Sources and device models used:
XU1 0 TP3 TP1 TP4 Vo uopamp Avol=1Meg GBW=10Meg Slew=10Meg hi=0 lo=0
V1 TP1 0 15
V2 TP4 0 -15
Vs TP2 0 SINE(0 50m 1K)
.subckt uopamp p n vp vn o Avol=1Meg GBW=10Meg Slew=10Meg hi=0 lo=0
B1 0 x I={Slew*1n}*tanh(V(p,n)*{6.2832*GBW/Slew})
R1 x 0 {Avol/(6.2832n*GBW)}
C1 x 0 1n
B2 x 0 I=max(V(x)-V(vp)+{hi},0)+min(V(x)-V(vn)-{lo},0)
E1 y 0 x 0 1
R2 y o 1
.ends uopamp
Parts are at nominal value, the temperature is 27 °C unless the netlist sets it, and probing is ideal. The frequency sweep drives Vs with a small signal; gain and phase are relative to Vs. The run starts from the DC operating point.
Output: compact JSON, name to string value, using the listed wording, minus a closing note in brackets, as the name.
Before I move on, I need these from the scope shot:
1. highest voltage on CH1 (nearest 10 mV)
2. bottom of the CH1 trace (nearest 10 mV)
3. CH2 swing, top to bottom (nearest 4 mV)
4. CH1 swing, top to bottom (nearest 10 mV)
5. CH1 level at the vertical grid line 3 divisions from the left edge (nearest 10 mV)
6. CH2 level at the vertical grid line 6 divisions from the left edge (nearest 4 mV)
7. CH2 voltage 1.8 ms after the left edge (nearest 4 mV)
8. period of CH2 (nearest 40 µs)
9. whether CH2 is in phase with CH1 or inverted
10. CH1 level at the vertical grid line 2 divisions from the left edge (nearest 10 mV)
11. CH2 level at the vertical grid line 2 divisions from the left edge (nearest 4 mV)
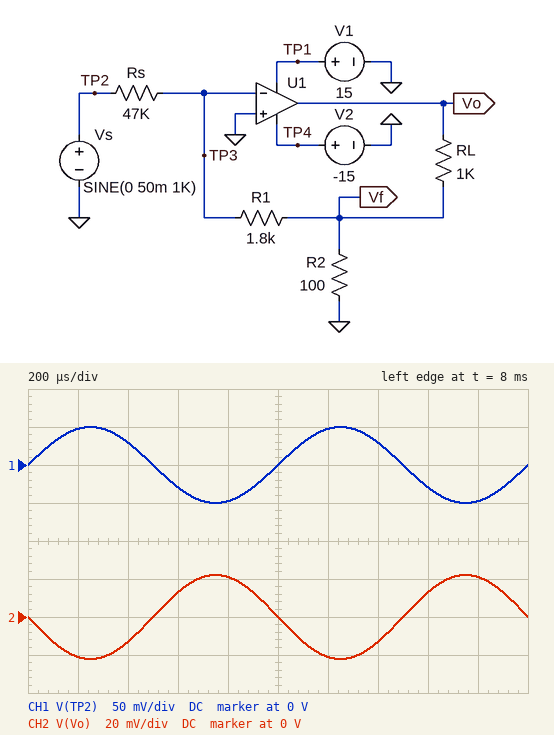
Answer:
{"highest voltage on CH1": "50 mV", "bottom of the CH1 trace": "-50 mV", "CH2 swing, top to bottom": "44 mV", "CH1 swing, top to bottom": "100 mV", "CH1 level at the vertical grid line 3 divisions from the left edge": "-30 mV", "CH2 level at the vertical grid line 6 divisions from the left edge": "-20 mV", "CH2 voltage 1.8 ms after the left edge": "20 mV", "period of CH2": "1.00 ms", "whether CH2 is in phase with CH1 or inverted": "inverted", "CH1 level at the vertical grid line 2 divisions from the left edge": "30 mV", "CH2 level at the vertical grid line 2 divisions from the left edge": "-12 mV"}
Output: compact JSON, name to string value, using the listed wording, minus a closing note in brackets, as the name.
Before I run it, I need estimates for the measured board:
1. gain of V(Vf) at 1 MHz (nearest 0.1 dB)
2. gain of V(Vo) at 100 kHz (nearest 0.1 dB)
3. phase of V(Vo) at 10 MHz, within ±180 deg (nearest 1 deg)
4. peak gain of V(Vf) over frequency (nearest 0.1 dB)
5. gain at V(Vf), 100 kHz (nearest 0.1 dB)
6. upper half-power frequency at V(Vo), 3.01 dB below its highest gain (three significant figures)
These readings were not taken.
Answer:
{"gain of V(Vf) at 1 MHz": "-32.0 dB", "gain of V(Vo) at 100 kHz": "-7.1 dB", "phase of V(Vo) at 10 MHz, within ±180 deg": "95 deg", "peak gain of V(Vf) over frequency": "-28.3 dB", "gain at V(Vf), 100 kHz": "-28.4 dB", "upper half-power frequency at V(Vo), 3.01 dB below its highest gain": "873 kHz"}
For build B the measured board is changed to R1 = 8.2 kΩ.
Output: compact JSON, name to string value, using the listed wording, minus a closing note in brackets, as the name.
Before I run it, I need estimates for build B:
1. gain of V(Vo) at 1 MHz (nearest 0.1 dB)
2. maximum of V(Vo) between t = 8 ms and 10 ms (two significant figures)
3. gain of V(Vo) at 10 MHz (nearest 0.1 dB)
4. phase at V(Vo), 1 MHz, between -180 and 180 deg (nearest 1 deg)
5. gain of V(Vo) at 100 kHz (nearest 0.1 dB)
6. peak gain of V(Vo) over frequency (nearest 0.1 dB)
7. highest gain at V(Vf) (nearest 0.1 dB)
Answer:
{"gain of V(Vo) at 1 MHz": "1.5 dB", "maximum of V(Vo) between t = 8 ms and 10 ms": "97 mV", "gain of V(Vo) at 10 MHz": "-16.5 dB", "phase at V(Vo), 1 MHz, between -180 and 180 deg": "128 deg", "gain of V(Vo) at 100 kHz": "5.7 dB", "peak gain of V(Vo) over frequency": "5.8 dB", "highest gain at V(Vf)": "-15.2 dB"}
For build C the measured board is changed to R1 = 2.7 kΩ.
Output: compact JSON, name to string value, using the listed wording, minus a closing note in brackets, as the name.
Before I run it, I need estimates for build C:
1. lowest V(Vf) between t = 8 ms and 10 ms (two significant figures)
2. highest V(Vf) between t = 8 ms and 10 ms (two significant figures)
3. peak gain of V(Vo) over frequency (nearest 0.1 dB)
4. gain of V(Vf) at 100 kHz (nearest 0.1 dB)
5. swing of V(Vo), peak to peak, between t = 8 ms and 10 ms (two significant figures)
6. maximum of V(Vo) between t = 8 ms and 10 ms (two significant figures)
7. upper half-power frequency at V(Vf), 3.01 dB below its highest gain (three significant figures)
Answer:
{"lowest V(Vf) between t = 8 ms and 10 ms": "-2.9 mV", "highest V(Vf) between t = 8 ms and 10 ms": "2.9 mV", "peak gain of V(Vo) over frequency": "-3.7 dB", "gain of V(Vf) at 100 kHz": "-24.9 dB", "swing of V(Vo), peak to peak, between t = 8 ms and 10 ms": "65 mV", "maximum of V(Vo) between t = 8 ms and 10 ms": "33 mV", "upper half-power frequency at V(Vf), 3.01 dB below its highest gain": "858 kHz"}
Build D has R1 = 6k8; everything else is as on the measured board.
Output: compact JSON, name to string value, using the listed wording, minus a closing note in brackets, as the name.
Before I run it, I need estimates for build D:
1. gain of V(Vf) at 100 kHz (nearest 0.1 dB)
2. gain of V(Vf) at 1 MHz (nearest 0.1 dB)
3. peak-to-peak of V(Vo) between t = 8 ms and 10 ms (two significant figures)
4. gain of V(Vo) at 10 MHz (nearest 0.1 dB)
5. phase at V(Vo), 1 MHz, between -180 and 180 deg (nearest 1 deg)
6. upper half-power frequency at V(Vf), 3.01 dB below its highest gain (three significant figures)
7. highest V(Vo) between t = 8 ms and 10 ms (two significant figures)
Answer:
{"gain of V(Vf) at 100 kHz": "-16.9 dB", "gain of V(Vf) at 1 MHz": "-20.9 dB", "peak-to-peak of V(Vo) between t = 8 ms and 10 ms": "160 mV", "gain of V(Vo) at 10 MHz": "-17.9 dB", "phase at V(Vo), 1 MHz, between -180 and 180 deg": "128 deg", "upper half-power frequency at V(Vf), 3.01 dB below its highest gain": "792 kHz", "highest V(Vo) between t = 8 ms and 10 ms": "81 mV"}
